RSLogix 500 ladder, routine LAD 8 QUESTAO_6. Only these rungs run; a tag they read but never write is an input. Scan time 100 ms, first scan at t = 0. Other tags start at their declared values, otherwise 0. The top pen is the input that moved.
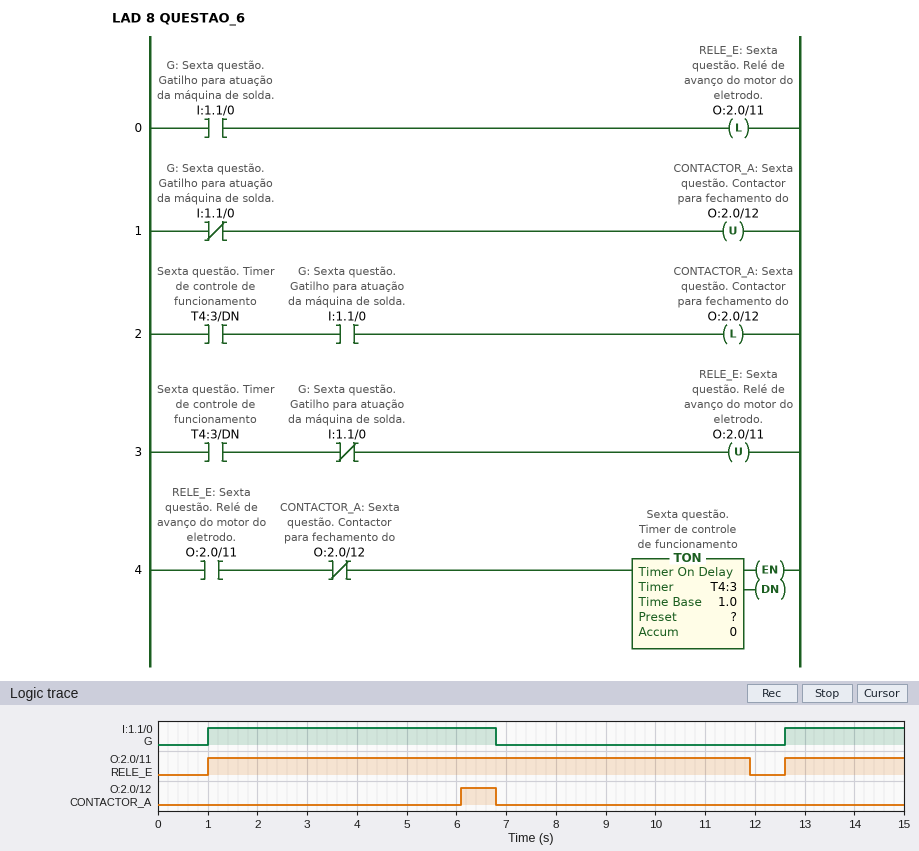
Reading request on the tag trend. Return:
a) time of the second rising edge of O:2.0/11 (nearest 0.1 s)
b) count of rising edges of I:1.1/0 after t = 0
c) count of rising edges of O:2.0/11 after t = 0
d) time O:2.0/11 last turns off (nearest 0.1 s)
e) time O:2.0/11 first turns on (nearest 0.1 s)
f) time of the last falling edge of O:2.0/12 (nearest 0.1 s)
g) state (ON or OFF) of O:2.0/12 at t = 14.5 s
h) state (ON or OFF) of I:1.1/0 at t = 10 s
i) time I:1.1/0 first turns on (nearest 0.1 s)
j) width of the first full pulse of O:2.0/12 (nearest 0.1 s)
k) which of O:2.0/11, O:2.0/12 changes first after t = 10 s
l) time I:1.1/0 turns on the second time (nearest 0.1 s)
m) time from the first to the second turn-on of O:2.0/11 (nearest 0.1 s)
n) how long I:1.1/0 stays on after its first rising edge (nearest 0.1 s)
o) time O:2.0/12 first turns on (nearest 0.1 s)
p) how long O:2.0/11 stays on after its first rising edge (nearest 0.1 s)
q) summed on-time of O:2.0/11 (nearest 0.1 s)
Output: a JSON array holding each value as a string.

["12.6 s", "2", "2", "11.9 s", "1.0 s", "6.8 s", "OFF", "OFF", "1.0 s", "0.7 s", "O:2.0/11", "12.6 s", "11.6 s", "5.8 s", "6.1 s", "10.9 s", "13.3 s"]
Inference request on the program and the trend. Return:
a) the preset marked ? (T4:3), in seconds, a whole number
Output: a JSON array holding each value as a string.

["5 s"]
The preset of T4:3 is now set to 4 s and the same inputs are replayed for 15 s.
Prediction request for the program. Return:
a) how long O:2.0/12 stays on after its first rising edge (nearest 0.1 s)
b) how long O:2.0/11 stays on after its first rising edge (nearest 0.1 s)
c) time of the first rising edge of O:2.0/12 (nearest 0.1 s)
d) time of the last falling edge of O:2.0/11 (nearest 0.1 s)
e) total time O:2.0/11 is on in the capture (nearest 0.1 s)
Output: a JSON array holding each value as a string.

["1.7 s", "9.9 s", "5.1 s", "10.9 s", "12.3 s"]
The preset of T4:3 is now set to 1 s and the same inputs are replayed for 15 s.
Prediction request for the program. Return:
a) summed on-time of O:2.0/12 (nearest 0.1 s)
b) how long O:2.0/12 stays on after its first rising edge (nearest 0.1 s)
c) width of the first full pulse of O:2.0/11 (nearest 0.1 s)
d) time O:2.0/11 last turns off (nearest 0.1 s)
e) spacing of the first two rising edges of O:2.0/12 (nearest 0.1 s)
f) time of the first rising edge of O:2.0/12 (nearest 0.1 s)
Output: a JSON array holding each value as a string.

["6.0 s", "4.7 s", "6.9 s", "7.9 s", "11.6 s", "2.1 s"]
